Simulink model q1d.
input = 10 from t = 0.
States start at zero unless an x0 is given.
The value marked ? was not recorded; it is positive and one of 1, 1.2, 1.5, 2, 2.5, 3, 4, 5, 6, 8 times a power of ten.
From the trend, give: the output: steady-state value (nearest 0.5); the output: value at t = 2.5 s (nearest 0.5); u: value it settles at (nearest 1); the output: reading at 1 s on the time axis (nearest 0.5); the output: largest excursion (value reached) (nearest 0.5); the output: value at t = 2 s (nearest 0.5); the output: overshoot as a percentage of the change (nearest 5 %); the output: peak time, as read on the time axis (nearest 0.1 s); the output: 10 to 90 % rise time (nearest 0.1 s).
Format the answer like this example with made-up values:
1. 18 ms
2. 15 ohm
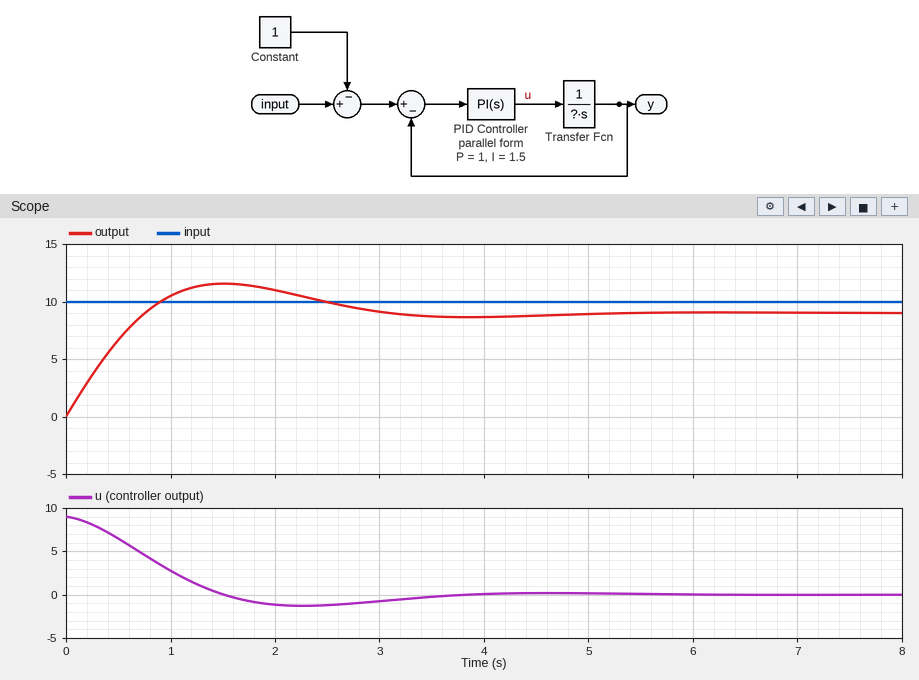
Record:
1. 9.0
2. 10.0
3. 0
4. 10.5
5. 11.5
6. 11.0
7. 30 %
8. 1.5 s
9. 0.6 s
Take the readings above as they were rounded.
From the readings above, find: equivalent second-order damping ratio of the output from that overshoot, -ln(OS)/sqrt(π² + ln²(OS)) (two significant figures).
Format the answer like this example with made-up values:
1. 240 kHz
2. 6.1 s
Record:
1. 0.36
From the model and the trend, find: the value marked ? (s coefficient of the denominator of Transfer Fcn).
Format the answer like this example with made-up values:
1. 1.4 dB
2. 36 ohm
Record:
1. 0.6
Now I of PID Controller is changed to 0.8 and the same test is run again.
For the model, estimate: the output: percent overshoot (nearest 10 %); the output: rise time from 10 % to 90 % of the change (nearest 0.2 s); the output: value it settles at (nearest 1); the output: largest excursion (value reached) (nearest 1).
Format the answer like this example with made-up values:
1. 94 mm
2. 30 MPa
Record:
1. 20 %
2. 0.8 s
3. 9
4. 11
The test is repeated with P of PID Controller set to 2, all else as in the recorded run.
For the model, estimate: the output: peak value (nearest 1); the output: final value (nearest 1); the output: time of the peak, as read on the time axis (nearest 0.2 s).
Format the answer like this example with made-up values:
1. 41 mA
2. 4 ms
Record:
1. 10
2. 9
3. 1.2 s
